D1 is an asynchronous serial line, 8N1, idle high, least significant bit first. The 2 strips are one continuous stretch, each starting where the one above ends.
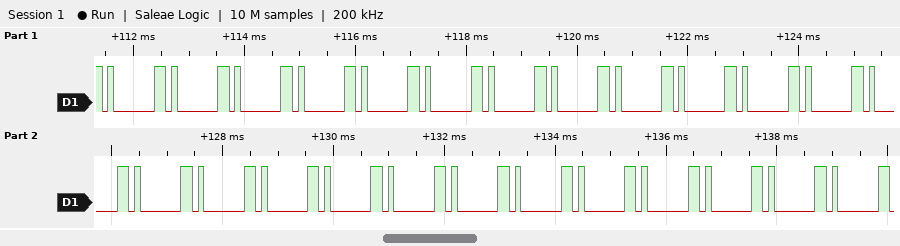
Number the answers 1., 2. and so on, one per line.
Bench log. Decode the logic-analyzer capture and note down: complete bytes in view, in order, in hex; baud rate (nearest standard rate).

1. 01 01 01 01 01 01 01 01 01 01 01 01 01 01 01 01 01 01 01 01 01 01 01 01 01
2. 9600 baud
